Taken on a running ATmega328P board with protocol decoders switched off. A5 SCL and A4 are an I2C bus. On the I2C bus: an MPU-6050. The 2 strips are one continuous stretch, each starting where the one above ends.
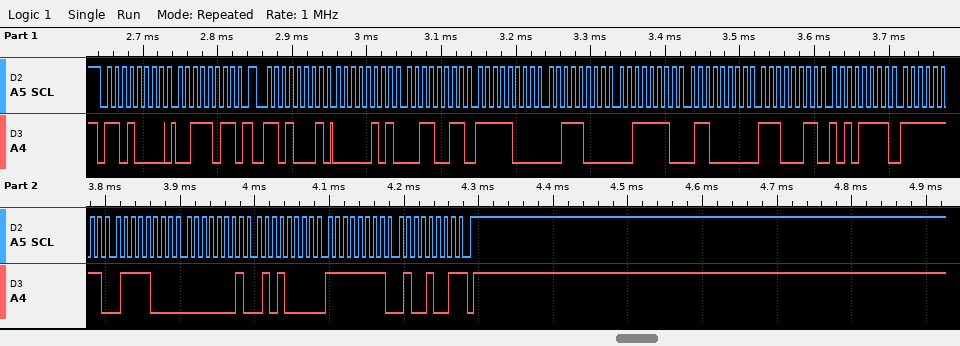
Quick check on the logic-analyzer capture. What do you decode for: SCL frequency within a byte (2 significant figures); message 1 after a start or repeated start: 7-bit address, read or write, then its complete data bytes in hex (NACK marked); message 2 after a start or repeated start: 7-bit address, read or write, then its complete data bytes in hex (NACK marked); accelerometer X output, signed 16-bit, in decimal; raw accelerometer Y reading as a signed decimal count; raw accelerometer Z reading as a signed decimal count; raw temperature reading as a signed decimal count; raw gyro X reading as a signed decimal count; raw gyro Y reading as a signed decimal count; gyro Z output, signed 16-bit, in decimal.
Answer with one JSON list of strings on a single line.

["100 kHz", "0x68 write: 3B", "0x68 read: 05 33 F8 38 3E 60 E3 AF FF 78 01 50 FF 49 NACK", "1331", "-1992", "15968", "-7249", "-136", "336", "-183"]
